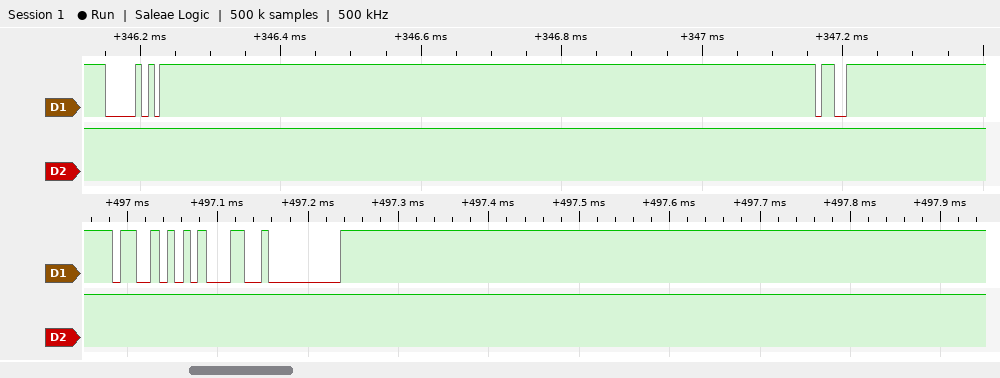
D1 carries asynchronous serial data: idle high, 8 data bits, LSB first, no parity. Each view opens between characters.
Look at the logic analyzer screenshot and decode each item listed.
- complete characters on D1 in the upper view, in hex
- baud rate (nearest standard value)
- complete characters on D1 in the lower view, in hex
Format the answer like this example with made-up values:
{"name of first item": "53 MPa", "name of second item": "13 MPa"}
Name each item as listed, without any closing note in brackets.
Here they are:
{"complete characters on D1 in the upper view, in hex": "50, F3", "baud rate": "115200 baud", "complete characters on D1 in the lower view, in hex": "53, 31, 00"}
